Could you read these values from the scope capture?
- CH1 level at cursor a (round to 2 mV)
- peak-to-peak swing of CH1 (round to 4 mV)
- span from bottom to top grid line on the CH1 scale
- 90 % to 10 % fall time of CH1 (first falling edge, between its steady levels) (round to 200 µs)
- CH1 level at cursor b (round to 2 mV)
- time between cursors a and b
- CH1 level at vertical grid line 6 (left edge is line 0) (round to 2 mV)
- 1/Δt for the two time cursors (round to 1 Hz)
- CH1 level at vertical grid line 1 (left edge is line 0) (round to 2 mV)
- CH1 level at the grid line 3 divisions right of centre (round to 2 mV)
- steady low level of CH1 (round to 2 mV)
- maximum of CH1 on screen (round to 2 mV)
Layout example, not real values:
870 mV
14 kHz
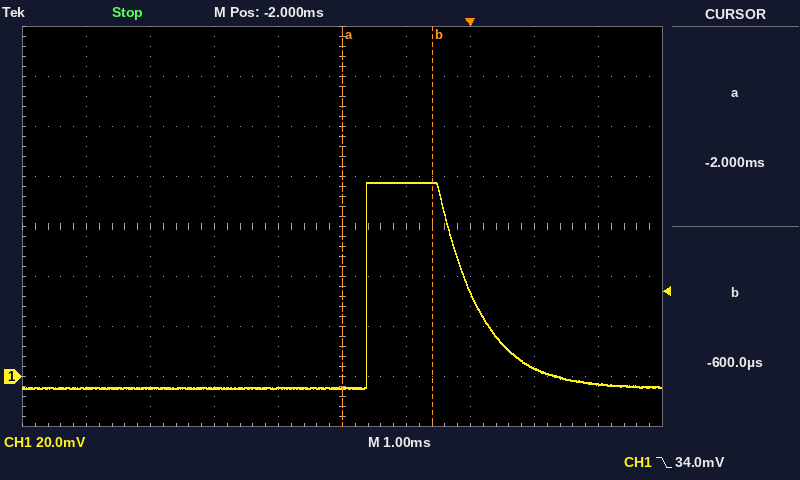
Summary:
-4 mV
84 mV
160 mV
1.4 ms
78 mV
1.4 ms
78 mV
714 Hz
-4 mV
4 mV
-4 mV
78 mV
